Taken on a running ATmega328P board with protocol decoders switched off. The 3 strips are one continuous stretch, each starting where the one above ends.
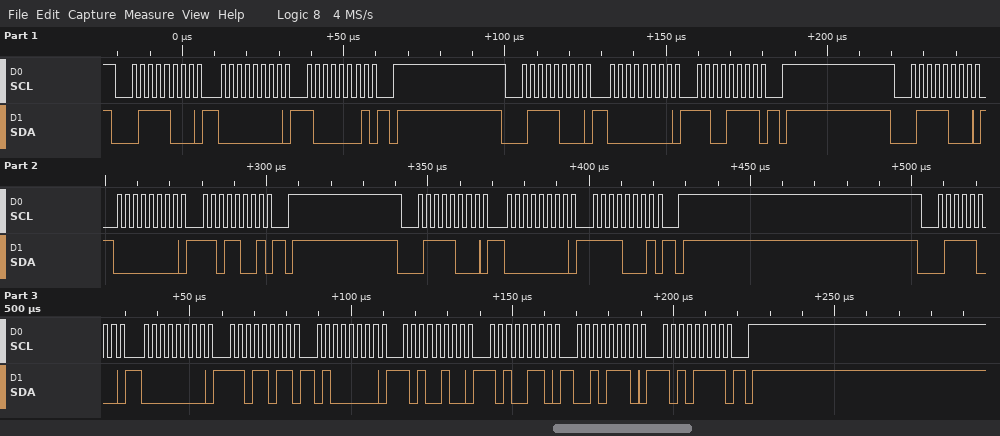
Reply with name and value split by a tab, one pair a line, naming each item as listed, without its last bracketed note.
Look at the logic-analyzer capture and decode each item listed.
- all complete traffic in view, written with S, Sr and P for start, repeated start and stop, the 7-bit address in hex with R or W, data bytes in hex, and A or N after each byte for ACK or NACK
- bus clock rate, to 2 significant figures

all complete traffic in view, written with S, Sr and P for start, repeated start and stop, the 7-bit address in hex with R or W, data bytes in hex, and A or N after each byte for ACK or NACK	S 3CW A 00 A 81 A P S 3CW A 00 A CF A P S 3CW A 00 A D9 A P S 3CW A 00 A F1 A P S 3CW A 00 A DB A 40 A A4 A A6 A 2E A AF A P
bus clock rate, to 2 significant figures	400 kHz
